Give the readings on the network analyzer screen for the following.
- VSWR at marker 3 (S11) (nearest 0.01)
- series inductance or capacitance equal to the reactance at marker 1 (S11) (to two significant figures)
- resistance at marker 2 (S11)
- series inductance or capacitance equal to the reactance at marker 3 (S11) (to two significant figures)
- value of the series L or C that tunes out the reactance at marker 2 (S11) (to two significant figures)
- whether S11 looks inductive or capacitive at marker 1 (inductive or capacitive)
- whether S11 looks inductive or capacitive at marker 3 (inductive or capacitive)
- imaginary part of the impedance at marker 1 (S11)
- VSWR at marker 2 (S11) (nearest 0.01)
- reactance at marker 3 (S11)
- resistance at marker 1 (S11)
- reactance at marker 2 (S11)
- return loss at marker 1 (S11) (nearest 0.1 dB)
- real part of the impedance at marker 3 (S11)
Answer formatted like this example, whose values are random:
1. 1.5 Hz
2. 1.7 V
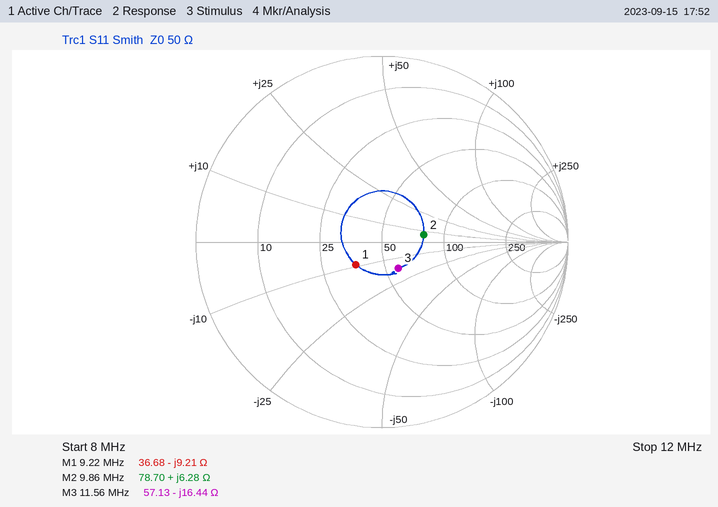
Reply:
1. 1.40
2. 1.9 nF
3. 78.70 Ω
4. 840 pF
5. 2.6 nF
6. capacitive
7. capacitive
8. -9.21 Ω
9. 1.59
10. -16.44 Ω
11. 36.68 Ω
12. +6.28 Ω
13. 14.6 dB
14. 57.13 Ω
